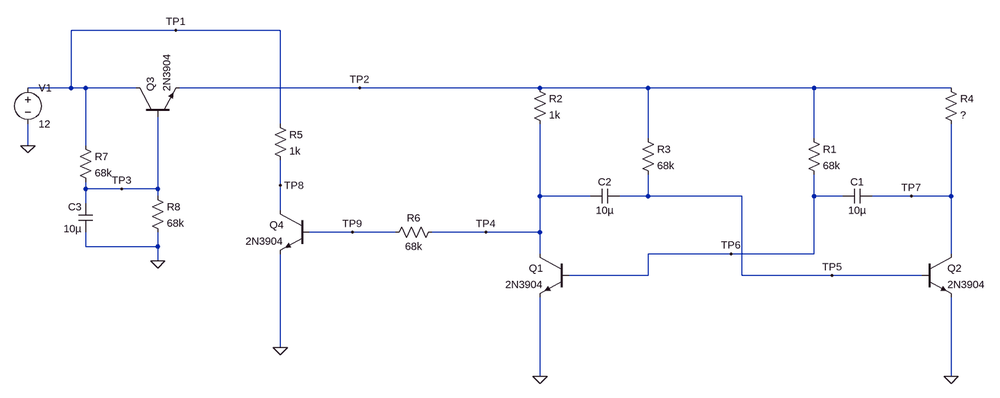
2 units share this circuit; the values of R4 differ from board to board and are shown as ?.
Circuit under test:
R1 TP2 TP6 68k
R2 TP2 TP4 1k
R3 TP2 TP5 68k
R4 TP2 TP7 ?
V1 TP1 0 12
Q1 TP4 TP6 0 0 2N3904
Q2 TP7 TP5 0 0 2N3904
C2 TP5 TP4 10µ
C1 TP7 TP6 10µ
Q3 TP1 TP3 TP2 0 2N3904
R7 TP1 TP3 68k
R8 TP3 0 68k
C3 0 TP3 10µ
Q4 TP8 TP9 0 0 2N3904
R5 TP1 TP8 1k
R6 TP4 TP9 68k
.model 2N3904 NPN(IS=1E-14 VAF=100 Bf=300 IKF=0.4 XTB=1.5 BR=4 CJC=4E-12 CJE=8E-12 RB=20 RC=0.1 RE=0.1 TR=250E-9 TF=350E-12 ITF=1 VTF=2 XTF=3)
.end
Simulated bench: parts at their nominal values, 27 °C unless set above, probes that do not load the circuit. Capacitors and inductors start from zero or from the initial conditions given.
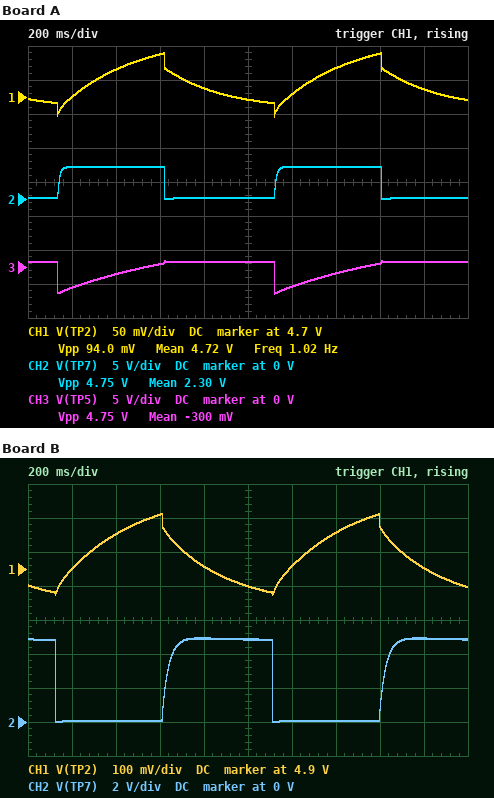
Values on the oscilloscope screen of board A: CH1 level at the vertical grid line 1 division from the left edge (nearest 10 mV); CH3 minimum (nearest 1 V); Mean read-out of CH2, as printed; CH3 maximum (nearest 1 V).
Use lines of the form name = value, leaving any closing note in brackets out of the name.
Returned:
CH1 level at the vertical grid line 1 division from the left edge = 4.70 V
CH3 minimum = -4 V
Mean read-out of CH2, as printed = 2.30 V
CH3 maximum = 1 V
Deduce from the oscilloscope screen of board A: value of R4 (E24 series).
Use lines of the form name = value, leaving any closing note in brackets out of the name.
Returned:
value of R4 = 820 Ω
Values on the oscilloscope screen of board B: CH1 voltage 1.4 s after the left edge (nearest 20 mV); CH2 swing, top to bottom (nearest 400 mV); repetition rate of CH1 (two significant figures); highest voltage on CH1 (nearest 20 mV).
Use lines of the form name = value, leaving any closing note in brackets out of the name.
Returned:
CH1 voltage 1.4 s after the left edge = 5.00 V
CH2 swing, top to bottom = 4.8 V
repetition rate of CH1 = 1.0 Hz
highest voltage on CH1 = 5.06 V
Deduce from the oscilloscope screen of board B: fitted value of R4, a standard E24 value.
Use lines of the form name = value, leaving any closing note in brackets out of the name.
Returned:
fitted value of R4, a standard E24 value = 3 kΩ
